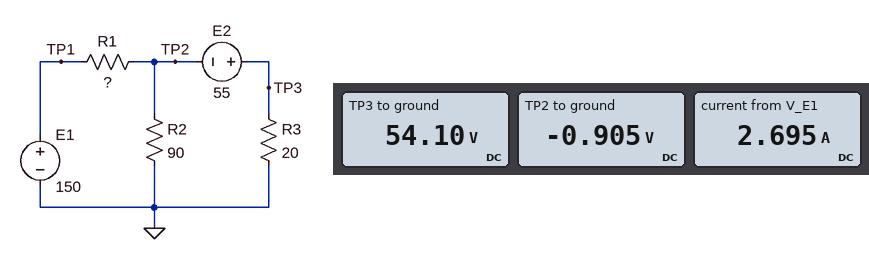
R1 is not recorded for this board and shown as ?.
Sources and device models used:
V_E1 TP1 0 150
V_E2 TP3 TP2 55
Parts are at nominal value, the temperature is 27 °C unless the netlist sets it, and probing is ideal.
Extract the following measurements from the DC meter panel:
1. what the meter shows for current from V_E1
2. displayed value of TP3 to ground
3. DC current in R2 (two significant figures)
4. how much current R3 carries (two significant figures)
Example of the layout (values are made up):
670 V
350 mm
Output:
2.695 A
54.10 V
10 mA
2.7 A
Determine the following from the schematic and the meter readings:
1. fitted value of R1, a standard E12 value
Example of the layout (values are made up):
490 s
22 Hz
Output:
56 Ω
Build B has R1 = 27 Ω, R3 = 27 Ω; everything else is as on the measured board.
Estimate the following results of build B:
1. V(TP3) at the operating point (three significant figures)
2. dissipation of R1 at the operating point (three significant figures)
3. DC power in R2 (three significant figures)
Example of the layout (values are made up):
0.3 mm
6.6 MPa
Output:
96.3 V
438 W
19.0 W
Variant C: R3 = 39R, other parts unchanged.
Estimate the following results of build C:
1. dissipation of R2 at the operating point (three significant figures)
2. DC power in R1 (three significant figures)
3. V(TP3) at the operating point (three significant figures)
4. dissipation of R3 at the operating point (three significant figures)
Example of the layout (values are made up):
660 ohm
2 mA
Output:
5.99 W
287 W
78.2 V
157 W
